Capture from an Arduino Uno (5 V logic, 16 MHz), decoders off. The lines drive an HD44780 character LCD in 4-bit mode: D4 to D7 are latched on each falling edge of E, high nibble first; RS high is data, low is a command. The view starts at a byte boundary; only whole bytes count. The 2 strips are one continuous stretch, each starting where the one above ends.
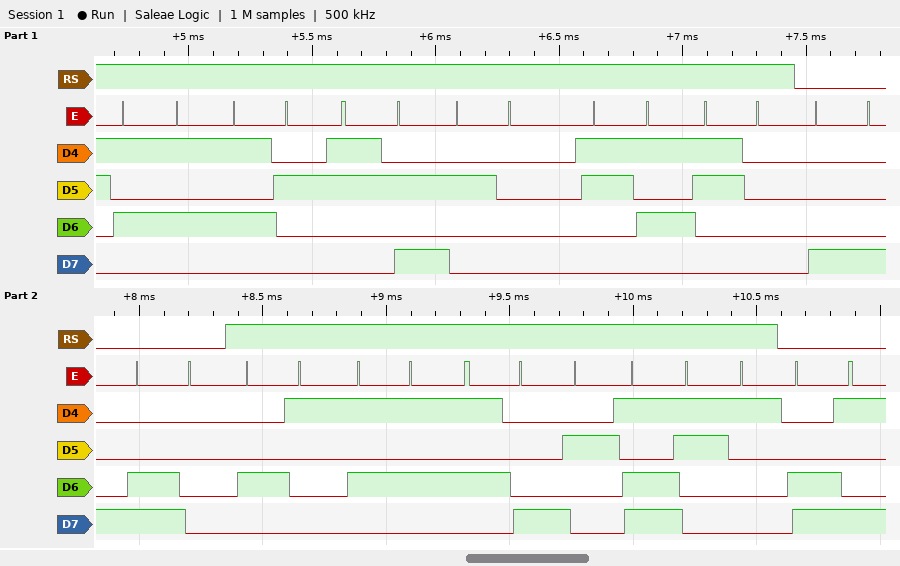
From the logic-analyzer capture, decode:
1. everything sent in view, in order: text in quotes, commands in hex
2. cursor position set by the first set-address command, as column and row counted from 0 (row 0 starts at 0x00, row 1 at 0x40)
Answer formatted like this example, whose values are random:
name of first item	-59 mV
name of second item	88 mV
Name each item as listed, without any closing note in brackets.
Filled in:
everything sent in view, in order: text in quotes, commands in hex	"UR: 50" 0x88 0xC0 "AUX-1" 0xC9
cursor position set by the first set-address command, as column and row counted from 0	column 8, row 0
